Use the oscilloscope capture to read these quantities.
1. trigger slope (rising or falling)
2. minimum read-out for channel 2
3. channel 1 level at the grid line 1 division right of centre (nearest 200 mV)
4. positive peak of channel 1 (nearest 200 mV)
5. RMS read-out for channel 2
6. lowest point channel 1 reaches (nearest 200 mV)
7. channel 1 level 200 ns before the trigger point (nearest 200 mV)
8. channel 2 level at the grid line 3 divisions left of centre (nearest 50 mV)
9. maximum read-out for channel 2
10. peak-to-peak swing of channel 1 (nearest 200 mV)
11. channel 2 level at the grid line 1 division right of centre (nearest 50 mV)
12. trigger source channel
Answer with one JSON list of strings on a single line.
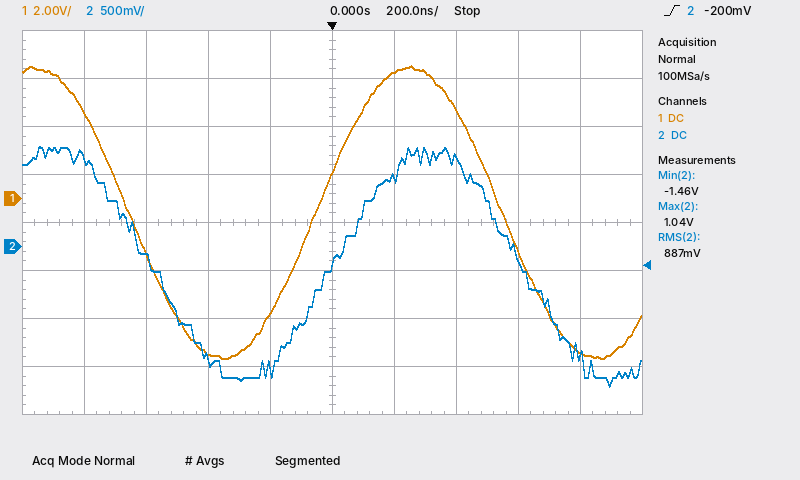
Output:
["rising", "-1.46 V", "5.2 V", "5.6 V", "887 mV", "-6.6 V", "-4.8 V", "-100 mV", "1.04 V", "12.2 V", "700 mV", "channel 2"]
